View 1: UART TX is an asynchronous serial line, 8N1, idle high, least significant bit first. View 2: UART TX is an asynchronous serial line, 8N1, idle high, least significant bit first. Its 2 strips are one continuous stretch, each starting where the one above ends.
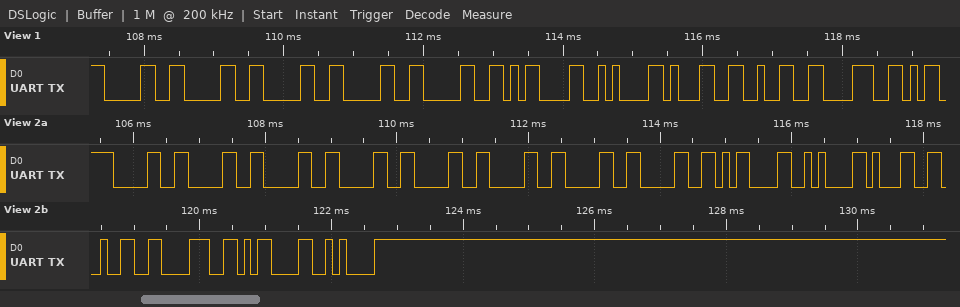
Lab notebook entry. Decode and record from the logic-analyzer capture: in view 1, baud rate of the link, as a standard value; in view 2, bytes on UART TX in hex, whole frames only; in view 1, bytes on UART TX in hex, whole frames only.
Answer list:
9600 baud
30 30 30 30 30 30 30 30 0D 0A 31 32 38 0D 0A
30 30 30 30 30 0D 0A 31 32 38
